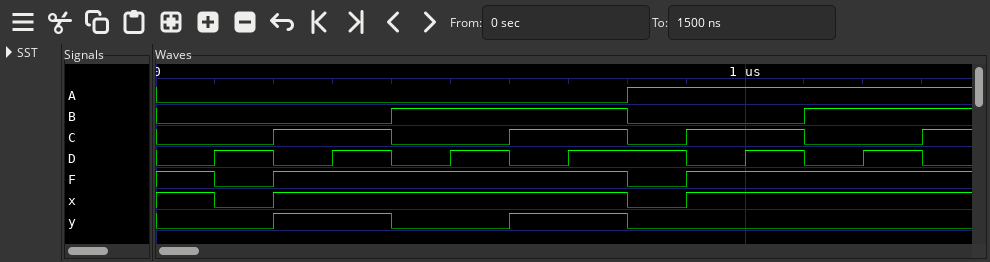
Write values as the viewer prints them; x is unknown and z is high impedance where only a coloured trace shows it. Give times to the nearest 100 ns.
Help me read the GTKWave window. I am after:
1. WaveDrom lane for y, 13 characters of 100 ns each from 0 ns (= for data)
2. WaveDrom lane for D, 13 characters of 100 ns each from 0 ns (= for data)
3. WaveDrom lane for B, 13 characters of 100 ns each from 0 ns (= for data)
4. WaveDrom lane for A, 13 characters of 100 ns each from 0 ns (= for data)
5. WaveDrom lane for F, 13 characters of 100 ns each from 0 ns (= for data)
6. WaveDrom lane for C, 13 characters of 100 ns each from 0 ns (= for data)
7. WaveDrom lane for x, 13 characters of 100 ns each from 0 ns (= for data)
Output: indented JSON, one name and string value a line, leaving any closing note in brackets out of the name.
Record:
{
  "WaveDrom lane for y, 13 characters of 100 ns each from 0 ns": "{name: 'y', wave: '0.1.0.1.0....'}",
  "WaveDrom lane for D, 13 characters of 100 ns each from 0 ns": "{name: 'D', wave: '01010101.0101'}",
  "WaveDrom lane for B, 13 characters of 100 ns each from 0 ns": "{name: 'B', wave: '0...1...0..1.'}",
  "WaveDrom lane for A, 13 characters of 100 ns each from 0 ns": "{name: 'A', wave: '0.......1....'}",
  "WaveDrom lane for F, 13 characters of 100 ns each from 0 ns": "{name: 'F', wave: '101.....01...'}",
  "WaveDrom lane for C, 13 characters of 100 ns each from 0 ns": "{name: 'C', wave: '0.1.0.1.01.0.'}",
  "WaveDrom lane for x, 13 characters of 100 ns each from 0 ns": "{name: 'x', wave: '101.....01...'}"
}
